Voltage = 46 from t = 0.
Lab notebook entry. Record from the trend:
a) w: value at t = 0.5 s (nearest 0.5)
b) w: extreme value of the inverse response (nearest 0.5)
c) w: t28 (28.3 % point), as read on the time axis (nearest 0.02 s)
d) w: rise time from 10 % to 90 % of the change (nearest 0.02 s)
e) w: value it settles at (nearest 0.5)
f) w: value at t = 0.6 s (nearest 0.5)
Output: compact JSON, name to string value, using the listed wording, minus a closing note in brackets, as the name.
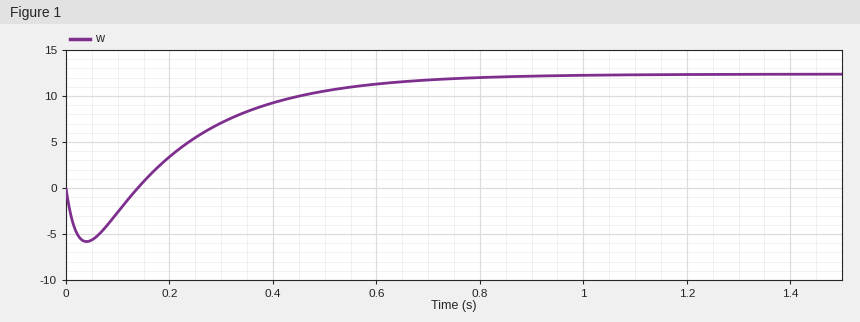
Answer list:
{"w: value at t = 0.5 s": "10.5", "w: extreme value of the inverse response": "-6.0", "w: t28 (28.3 % point), as read on the time axis": "0.20 s", "w: rise time from 10 % to 90 % of the change": "0.42 s", "w: value it settles at": "12.5", "w: value at t = 0.6 s": "11.5"}
